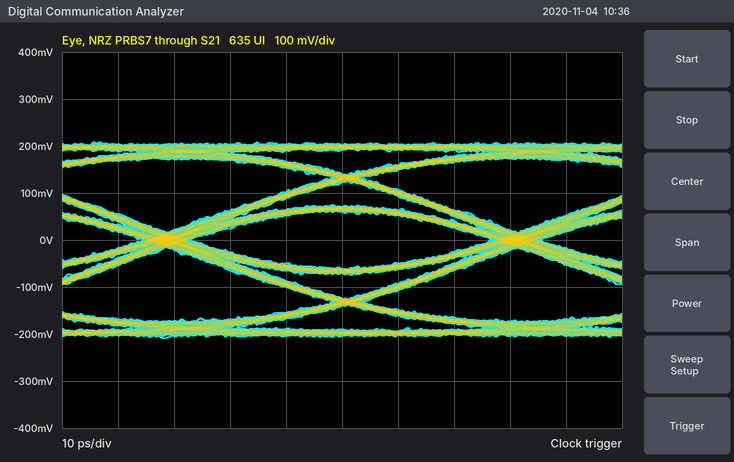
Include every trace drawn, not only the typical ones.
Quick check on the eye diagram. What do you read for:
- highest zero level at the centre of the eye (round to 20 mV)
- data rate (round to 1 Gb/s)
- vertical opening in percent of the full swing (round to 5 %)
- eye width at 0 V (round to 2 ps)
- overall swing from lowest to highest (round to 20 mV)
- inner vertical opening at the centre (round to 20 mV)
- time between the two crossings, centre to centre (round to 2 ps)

-60 mV
16 Gb/s
30 %
54 ps
420 mV
120 mV
62 ps
